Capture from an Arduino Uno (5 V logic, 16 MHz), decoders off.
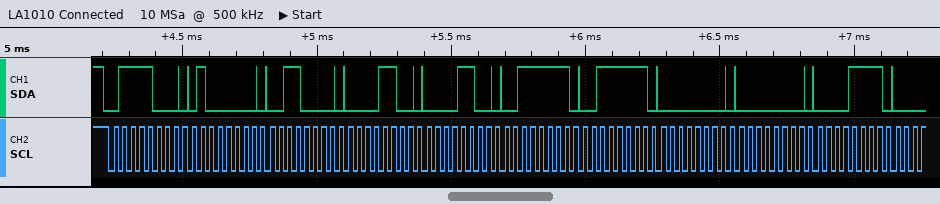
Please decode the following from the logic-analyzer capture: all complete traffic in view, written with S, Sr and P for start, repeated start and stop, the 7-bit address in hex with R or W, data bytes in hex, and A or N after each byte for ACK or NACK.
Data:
S 3CW A 40 A 30 A 0C A 0C A 3F A 3F A 00 A 00 A 0F A
